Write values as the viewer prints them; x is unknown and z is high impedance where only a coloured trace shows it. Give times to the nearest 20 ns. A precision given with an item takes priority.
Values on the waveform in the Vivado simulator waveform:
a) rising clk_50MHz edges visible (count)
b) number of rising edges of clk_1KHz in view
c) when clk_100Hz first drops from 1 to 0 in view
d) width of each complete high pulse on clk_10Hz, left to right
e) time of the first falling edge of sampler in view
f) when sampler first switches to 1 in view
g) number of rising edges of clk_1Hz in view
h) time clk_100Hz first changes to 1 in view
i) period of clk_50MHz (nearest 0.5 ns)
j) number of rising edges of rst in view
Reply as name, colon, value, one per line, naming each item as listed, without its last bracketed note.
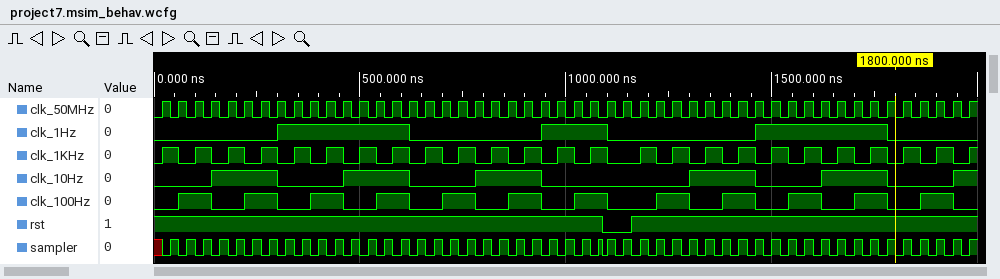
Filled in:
rising clk_50MHz edges visible: 50
number of rising edges of clk_1KHz in view: 25
when clk_100Hz first drops from 1 to 0 in view: 140 ns
width of each complete high pulse on clk_10Hz, left to right: 160 ns, 160 ns, 160 ns, 160 ns, 160 ns
time of the first falling edge of sampler in view: 60 ns
when sampler first switches to 1 in view: 40 ns
number of rising edges of clk_1Hz in view: 3
time clk_100Hz first changes to 1 in view: 60 ns
period of clk_50MHz: 40 ns
number of rising edges of rst in view: 1
